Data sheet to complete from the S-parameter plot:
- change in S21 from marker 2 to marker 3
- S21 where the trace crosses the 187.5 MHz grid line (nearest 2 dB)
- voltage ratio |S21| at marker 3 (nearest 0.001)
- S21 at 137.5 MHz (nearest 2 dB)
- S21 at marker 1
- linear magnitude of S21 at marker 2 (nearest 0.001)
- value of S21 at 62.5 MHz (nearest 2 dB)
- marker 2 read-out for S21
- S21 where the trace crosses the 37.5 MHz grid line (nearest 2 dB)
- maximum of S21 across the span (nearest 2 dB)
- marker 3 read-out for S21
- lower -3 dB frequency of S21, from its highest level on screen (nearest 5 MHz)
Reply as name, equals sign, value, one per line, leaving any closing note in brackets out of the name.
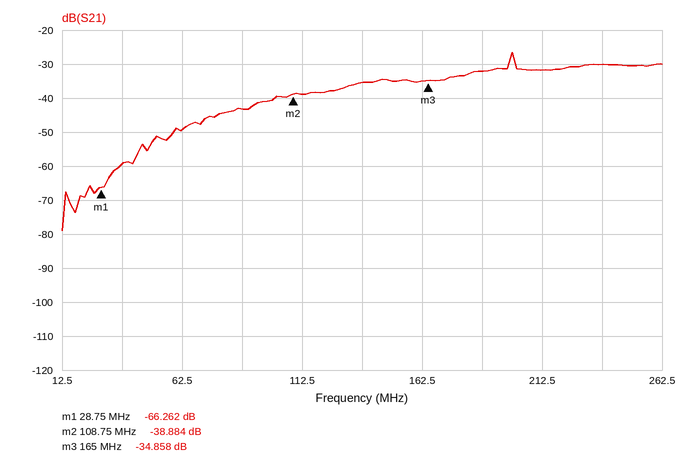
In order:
change in S21 from marker 2 to marker 3 = 4.026 dB
S21 where the trace crosses the 187.5 MHz grid line = -32 dB
voltage ratio |S21| at marker 3 = 0.018
S21 at 137.5 MHz = -36 dB
S21 at marker 1 = -66.262 dB
linear magnitude of S21 at marker 2 = 0.011
value of S21 at 62.5 MHz = -50 dB
marker 2 read-out for S21 = -38.884 dB
S21 where the trace crosses the 37.5 MHz grid line = -60 dB
maximum of S21 across the span = -26 dB
marker 3 read-out for S21 = -34.858 dB
lower -3 dB frequency of S21, from its highest level on screen = 200 MHz
